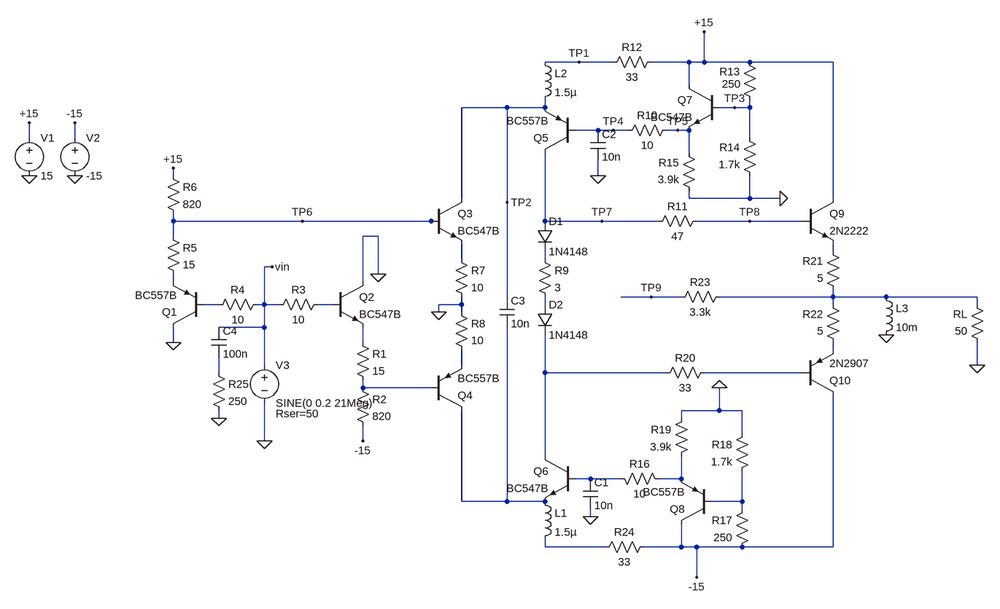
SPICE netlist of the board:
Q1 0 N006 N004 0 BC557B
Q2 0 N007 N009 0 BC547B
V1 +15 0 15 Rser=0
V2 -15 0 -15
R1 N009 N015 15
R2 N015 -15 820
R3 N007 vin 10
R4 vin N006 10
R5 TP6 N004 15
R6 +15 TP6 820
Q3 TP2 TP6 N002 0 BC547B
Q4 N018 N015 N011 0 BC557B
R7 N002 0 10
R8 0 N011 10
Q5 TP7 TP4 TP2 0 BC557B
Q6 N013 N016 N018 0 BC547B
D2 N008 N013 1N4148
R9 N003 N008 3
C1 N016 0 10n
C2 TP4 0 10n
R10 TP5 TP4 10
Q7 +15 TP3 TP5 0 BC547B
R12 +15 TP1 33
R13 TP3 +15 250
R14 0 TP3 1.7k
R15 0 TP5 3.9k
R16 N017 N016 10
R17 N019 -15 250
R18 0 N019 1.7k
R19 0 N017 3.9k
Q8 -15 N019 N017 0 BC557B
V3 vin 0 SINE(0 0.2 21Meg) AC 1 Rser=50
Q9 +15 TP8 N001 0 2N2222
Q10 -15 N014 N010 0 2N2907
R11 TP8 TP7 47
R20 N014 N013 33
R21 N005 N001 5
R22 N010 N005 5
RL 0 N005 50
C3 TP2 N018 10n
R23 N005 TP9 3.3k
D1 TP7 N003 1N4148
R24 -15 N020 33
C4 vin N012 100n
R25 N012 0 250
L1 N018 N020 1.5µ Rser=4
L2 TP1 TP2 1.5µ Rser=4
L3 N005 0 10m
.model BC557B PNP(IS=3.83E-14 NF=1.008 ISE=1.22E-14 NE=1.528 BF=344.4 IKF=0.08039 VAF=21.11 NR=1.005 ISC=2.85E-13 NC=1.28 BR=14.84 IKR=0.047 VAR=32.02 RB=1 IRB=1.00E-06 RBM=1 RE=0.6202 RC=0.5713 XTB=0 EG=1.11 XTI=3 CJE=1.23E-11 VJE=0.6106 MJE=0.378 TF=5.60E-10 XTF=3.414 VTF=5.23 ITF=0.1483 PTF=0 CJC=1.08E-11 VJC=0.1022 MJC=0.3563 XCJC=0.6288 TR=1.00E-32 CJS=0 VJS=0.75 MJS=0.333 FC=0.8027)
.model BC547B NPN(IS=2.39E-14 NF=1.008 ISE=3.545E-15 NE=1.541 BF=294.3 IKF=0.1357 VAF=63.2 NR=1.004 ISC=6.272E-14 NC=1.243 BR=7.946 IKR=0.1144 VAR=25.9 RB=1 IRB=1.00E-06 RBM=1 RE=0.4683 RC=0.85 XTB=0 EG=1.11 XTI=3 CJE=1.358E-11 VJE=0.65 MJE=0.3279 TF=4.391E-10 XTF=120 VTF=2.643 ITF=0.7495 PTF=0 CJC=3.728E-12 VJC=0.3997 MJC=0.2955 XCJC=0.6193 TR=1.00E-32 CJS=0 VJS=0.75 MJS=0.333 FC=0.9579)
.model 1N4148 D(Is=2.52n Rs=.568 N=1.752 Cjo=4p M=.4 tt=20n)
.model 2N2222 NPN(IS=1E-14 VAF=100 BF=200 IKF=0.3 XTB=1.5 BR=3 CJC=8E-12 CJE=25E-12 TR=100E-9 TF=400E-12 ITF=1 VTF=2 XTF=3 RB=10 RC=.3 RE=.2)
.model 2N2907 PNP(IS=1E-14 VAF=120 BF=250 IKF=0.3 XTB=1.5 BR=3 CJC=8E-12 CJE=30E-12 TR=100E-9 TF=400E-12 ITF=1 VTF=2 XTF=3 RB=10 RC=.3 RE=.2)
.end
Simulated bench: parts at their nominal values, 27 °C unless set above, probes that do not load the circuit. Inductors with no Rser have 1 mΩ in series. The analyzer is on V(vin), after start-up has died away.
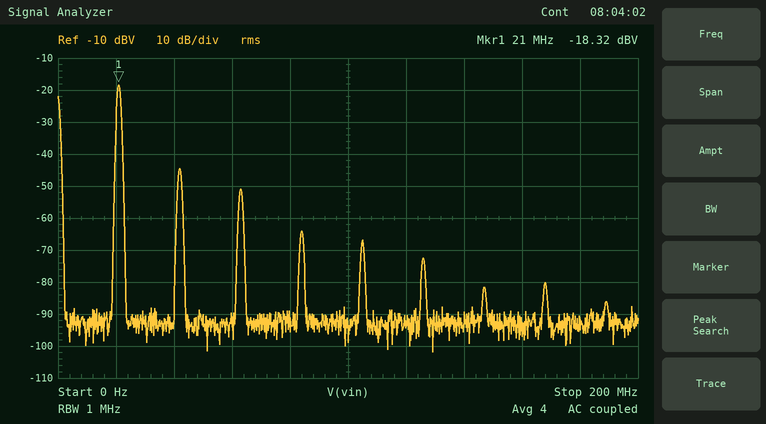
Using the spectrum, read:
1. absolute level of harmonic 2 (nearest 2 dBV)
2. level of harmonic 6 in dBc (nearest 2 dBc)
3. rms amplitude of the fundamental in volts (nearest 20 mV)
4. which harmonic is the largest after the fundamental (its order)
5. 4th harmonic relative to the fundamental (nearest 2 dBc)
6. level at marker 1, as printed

-44 dBV
-54 dBc
120 mV
2
-46 dBc
-18.32 dBV
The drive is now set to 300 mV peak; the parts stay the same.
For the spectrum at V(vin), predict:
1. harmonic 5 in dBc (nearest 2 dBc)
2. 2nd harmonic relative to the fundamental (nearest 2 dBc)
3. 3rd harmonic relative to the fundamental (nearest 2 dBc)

-42 dBc
-22 dBc
-30 dBc
